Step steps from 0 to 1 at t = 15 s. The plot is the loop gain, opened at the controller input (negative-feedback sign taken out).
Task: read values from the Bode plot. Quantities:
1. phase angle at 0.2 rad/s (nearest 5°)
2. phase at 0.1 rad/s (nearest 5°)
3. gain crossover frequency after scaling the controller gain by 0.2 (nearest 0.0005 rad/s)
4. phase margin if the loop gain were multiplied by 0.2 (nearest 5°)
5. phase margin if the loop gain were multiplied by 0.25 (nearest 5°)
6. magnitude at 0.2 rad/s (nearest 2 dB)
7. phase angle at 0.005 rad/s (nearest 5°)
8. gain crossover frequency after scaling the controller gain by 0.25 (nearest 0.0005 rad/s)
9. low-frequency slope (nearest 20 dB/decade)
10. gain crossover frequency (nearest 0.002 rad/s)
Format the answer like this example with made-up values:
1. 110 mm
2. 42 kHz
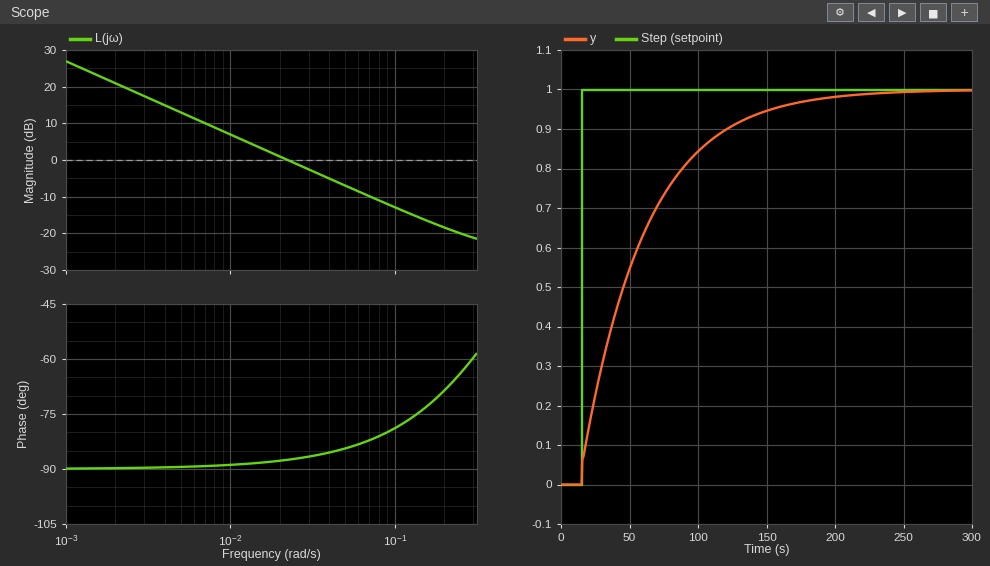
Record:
1. -70°
2. -80°
3. 0.0045 rad/s
4. 90°
5. 90°
6. -18 dB
7. -90°
8. 0.0055 rad/s
9. -20 dB/decade
10. 0.022 rad/s
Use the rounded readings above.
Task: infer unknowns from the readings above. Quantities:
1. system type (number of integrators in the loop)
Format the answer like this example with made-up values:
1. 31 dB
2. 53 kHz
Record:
1. 1
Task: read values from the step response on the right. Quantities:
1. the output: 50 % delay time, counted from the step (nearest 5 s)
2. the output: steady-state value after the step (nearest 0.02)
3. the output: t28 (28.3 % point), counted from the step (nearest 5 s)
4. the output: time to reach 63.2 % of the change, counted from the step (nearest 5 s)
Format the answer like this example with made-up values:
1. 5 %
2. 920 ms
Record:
1. 30 s
2. 1.00
3. 15 s
4. 45 s
